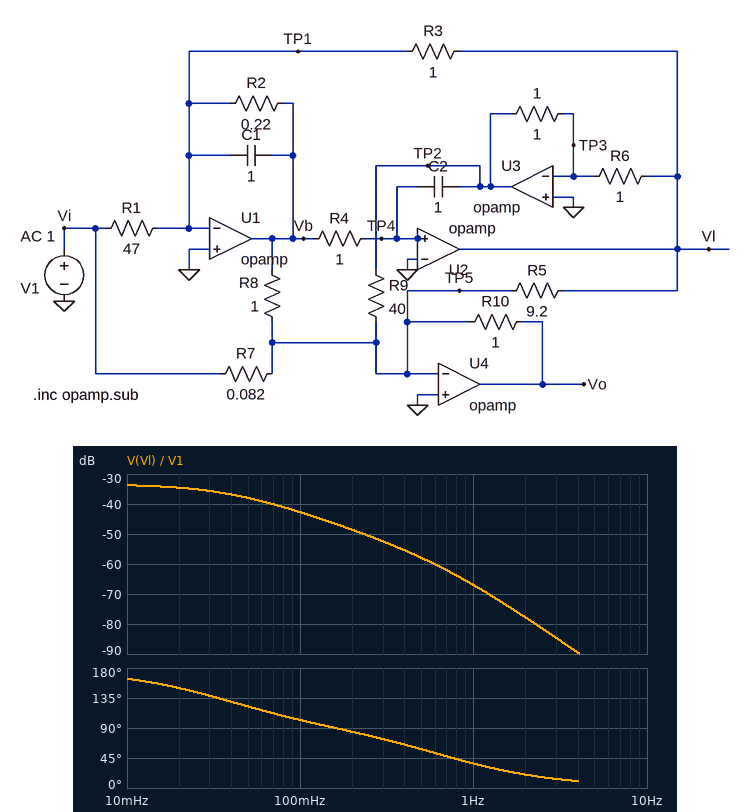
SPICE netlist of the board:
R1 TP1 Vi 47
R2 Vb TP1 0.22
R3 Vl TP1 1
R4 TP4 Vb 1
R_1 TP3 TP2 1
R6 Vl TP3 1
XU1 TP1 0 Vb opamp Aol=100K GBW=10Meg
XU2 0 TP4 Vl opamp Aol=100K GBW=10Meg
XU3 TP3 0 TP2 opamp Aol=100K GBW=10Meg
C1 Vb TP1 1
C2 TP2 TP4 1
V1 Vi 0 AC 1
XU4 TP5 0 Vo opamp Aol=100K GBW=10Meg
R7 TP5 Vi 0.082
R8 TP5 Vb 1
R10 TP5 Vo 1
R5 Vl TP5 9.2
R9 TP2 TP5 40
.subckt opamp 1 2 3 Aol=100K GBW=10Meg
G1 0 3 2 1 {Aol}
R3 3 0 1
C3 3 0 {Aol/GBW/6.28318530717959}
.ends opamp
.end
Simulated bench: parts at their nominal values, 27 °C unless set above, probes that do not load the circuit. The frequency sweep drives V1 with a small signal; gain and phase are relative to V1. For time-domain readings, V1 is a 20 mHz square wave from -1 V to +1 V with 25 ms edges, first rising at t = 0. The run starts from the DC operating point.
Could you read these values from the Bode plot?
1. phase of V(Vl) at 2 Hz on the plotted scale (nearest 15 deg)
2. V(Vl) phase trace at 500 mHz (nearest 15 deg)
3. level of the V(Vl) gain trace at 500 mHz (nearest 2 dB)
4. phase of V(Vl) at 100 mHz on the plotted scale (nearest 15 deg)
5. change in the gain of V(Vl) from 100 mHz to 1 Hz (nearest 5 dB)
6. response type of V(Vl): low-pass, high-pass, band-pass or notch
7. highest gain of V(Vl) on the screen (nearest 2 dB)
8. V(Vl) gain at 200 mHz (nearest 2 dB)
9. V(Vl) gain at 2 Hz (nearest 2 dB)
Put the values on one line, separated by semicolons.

15 deg; 60 deg; -58 dB; 105 deg; -25 dB; low-pass; -34 dB; -48 dB; -78 dB
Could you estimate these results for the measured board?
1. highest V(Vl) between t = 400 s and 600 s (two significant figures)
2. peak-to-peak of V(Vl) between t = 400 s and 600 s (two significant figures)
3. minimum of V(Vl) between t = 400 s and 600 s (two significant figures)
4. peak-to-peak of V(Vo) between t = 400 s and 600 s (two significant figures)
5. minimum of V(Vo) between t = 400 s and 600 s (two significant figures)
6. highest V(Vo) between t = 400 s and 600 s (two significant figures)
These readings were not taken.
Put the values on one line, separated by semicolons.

21 mV; 42 mV; -21 mV; 24 V; -12 V; 12 V
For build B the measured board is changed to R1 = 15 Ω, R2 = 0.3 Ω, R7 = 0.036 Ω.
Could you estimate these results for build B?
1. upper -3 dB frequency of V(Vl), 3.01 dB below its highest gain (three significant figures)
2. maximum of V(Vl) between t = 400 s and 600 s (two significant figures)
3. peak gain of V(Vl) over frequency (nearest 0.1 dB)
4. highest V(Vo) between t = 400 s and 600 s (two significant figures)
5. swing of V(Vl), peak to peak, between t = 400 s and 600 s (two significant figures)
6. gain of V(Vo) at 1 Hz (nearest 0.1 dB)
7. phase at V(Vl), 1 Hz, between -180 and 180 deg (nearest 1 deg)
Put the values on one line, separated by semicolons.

52.4 mHz; 67 mV; -23.5 dB; 28 V; 130 mV; 28.9 dB; 29 deg
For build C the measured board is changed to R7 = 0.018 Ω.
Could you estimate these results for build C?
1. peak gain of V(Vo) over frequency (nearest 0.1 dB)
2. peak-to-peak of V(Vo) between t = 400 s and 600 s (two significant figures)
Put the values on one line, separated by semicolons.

34.9 dB; 110 V
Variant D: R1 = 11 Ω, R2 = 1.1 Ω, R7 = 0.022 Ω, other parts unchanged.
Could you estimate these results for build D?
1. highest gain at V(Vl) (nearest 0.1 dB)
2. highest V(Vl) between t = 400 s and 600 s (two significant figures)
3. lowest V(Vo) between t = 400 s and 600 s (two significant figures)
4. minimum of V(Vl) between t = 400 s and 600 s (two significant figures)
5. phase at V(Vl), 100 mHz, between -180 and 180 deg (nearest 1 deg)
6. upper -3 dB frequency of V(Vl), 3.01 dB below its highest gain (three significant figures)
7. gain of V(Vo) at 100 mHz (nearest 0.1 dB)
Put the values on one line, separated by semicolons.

-19.0 dB; 130 mV; -45 V; -130 mV; 137 deg; 188 mHz; 33.1 dB
